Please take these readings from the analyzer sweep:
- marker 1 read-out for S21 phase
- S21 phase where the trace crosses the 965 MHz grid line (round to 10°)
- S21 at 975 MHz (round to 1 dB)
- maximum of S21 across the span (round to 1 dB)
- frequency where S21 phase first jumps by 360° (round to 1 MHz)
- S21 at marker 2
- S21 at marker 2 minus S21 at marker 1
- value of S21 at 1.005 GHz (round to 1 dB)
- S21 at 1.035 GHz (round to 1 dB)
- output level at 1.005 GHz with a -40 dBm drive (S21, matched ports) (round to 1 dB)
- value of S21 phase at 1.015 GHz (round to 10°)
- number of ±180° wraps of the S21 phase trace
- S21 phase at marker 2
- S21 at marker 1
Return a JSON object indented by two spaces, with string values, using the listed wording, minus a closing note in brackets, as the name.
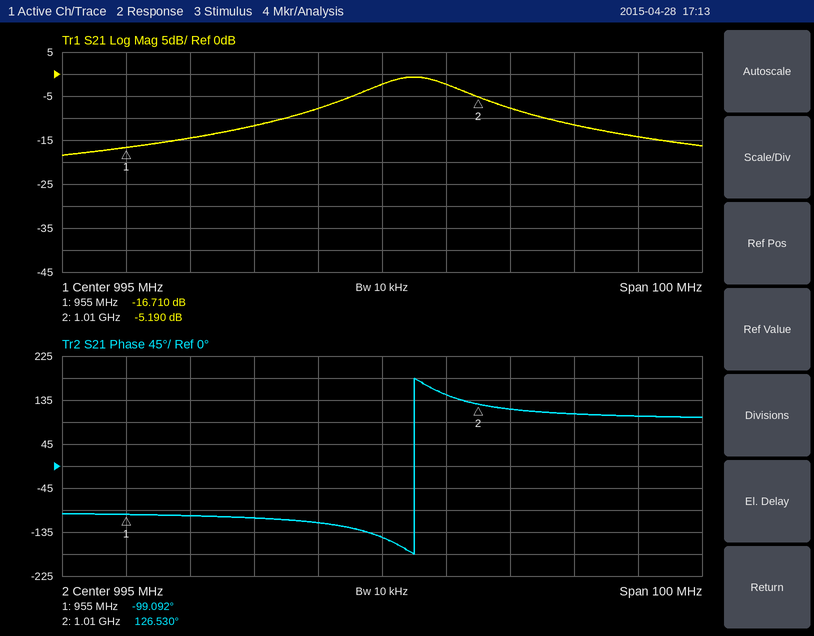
{
  "marker 1 read-out for S21 phase": "-99.092°",
  "S21 phase where the trace crosses the 965 MHz grid line": "-100°",
  "S21 at 975 MHz": "-12 dB",
  "maximum of S21 across the span": "-1 dB",
  "frequency where S21 phase first jumps by 360°": "1.000 GHz",
  "S21 at marker 2": "-5.190 dB",
  "S21 at marker 2 minus S21 at marker 1": "11.520 dB",
  "value of S21 at 1.005 GHz": "-2 dB",
  "S21 at 1.035 GHz": "-14 dB",
  "output level at 1.005 GHz with a -40 dBm drive (S21, matched ports)": "-42 dBm",
  "value of S21 phase at 1.015 GHz": "120°",
  "number of ±180° wraps of the S21 phase trace": "1",
  "S21 phase at marker 2": "126.530°",
  "S21 at marker 1": "-16.710 dB"
}
